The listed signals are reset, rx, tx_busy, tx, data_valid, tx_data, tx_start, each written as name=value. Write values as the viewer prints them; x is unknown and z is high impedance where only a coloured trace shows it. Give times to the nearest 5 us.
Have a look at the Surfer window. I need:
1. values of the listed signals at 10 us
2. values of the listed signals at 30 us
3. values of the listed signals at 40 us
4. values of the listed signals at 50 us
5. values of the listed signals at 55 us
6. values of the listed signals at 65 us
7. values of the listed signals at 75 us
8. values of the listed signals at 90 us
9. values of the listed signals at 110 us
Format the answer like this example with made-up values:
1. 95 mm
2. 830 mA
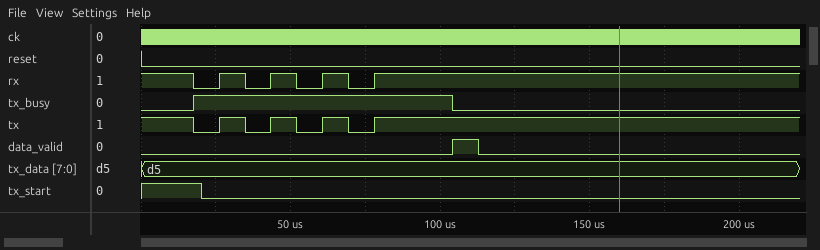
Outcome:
1. reset=0, rx=1, tx_busy=0, tx=1, data_valid=0, tx_data=d5, tx_start=1
2. reset=0, rx=1, tx_busy=1, tx=1, data_valid=0, tx_data=d5, tx_start=0
3. reset=0, rx=0, tx_busy=1, tx=0, data_valid=0, tx_data=d5, tx_start=0
4. reset=0, rx=1, tx_busy=1, tx=1, data_valid=0, tx_data=d5, tx_start=0
5. reset=0, rx=0, tx_busy=1, tx=0, data_valid=0, tx_data=d5, tx_start=0
6. reset=0, rx=1, tx_busy=1, tx=1, data_valid=0, tx_data=d5, tx_start=0
7. reset=0, rx=0, tx_busy=1, tx=0, data_valid=0, tx_data=d5, tx_start=0
8. reset=0, rx=1, tx_busy=1, tx=1, data_valid=0, tx_data=d5, tx_start=0
9. reset=0, rx=1, tx_busy=0, tx=1, data_valid=1, tx_data=d5, tx_start=0
